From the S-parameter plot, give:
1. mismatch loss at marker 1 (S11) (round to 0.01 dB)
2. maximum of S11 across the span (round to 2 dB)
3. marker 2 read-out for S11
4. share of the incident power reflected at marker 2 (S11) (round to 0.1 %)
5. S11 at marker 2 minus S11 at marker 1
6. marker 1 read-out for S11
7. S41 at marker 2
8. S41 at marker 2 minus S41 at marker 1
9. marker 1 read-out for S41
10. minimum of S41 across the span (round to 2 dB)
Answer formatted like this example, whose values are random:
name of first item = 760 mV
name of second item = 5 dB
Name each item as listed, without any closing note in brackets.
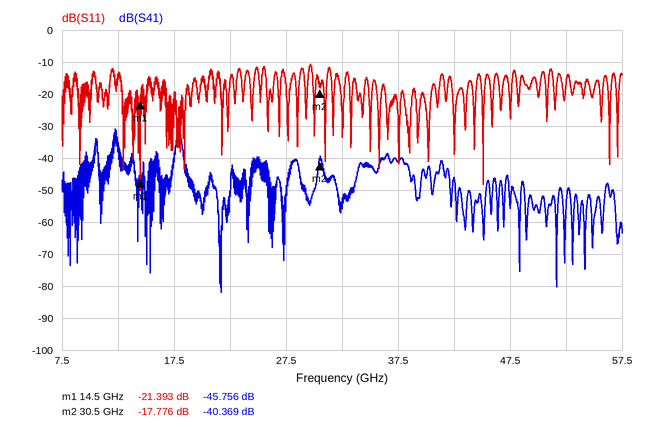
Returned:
mismatch loss at marker 1 (S11) = 0.03 dB
maximum of S11 across the span = -10 dB
marker 2 read-out for S11 = -17.776 dB
share of the incident power reflected at marker 2 (S11) = 1.7 %
S11 at marker 2 minus S11 at marker 1 = 3.617 dB
marker 1 read-out for S11 = -21.393 dB
S41 at marker 2 = -40.369 dB
S41 at marker 2 minus S41 at marker 1 = 5.387 dB
marker 1 read-out for S41 = -45.756 dB
minimum of S41 across the span = -82 dB
